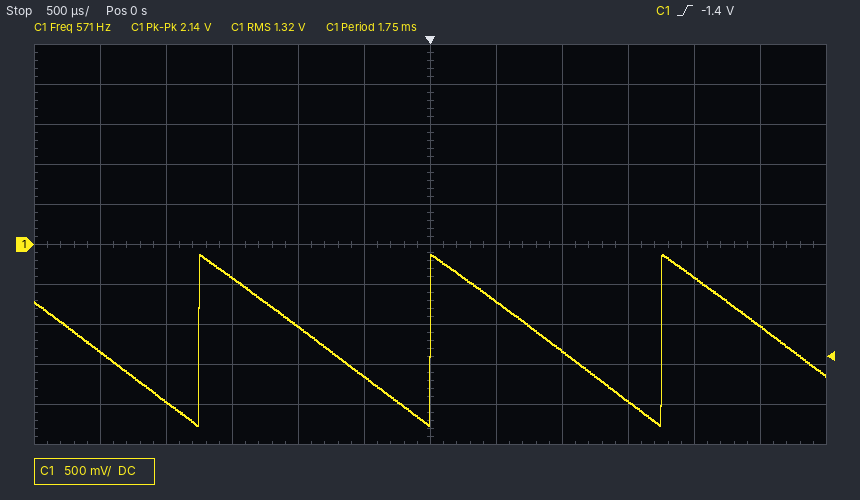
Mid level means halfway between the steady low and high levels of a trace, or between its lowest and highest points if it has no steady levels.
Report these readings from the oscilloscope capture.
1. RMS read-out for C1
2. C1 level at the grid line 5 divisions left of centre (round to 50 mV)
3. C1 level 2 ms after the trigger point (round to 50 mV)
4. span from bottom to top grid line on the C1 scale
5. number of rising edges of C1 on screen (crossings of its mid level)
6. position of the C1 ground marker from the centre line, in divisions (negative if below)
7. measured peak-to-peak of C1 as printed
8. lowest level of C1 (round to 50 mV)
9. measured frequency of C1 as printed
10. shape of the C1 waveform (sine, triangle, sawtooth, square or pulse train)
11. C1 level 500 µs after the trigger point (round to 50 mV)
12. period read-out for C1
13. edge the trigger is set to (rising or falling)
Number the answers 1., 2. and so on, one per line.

1. 1.32 V
2. -1.35 V
3. -400 mV
4. 5 V
5. 3
6. 0.0 div
7. 2.14 V
8. -2.25 V
9. 571 Hz
10. sawtooth
11. -700 mV
12. 1.75 ms
13. rising
